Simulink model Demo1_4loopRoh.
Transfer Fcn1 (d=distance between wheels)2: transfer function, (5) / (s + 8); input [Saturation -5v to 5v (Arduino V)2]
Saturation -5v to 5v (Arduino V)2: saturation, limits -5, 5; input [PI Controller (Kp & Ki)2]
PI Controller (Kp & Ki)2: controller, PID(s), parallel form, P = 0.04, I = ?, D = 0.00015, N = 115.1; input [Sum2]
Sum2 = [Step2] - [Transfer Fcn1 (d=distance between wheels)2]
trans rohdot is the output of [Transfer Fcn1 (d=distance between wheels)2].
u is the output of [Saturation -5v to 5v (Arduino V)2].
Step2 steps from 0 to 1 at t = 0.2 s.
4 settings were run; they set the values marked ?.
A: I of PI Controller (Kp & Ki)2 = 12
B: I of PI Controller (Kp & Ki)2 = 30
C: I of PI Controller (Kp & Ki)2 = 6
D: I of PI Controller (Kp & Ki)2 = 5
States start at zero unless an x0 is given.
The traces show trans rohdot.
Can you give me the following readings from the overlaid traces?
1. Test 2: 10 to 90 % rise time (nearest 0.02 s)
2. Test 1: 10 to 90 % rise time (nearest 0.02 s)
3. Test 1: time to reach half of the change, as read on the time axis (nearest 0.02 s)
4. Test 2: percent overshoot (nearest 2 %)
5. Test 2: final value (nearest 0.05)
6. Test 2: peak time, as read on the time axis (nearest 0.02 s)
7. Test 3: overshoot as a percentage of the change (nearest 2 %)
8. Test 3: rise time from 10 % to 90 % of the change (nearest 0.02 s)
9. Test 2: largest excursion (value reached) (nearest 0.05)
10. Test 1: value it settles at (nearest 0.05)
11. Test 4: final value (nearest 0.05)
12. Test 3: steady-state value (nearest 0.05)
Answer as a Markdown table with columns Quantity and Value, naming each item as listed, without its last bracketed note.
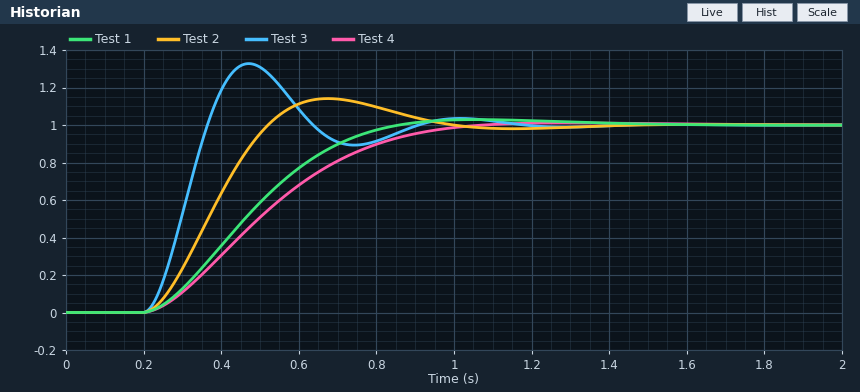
| Quantity | Value |
|---|---|
| Test 2: 10 to 90 % rise time | 0.22 s |
| Test 1: 10 to 90 % rise time | 0.42 s |
| Test 1: time to reach half of the change, as read on the time axis | 0.46 s |
| Test 2: percent overshoot | 14 % |
| Test 2: final value | 1.00 |
| Test 2: peak time, as read on the time axis | 0.68 s |
| Test 3: overshoot as a percentage of the change | 32 % |
| Test 3: rise time from 10 % to 90 % of the change | 0.12 s |
| Test 2: largest excursion (value reached) | 1.15 |
| Test 1: value it settles at | 1.00 |
| Test 4: final value | 1.00 |
| Test 3: steady-state value | 1.00 |
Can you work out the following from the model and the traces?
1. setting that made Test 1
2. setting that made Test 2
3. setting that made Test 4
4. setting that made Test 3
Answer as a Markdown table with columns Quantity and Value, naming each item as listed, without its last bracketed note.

| Quantity | Value |
|---|---|
| setting that made Test 1 | C |
| setting that made Test 2 | A |
| setting that made Test 4 | D |
| setting that made Test 3 | B |
